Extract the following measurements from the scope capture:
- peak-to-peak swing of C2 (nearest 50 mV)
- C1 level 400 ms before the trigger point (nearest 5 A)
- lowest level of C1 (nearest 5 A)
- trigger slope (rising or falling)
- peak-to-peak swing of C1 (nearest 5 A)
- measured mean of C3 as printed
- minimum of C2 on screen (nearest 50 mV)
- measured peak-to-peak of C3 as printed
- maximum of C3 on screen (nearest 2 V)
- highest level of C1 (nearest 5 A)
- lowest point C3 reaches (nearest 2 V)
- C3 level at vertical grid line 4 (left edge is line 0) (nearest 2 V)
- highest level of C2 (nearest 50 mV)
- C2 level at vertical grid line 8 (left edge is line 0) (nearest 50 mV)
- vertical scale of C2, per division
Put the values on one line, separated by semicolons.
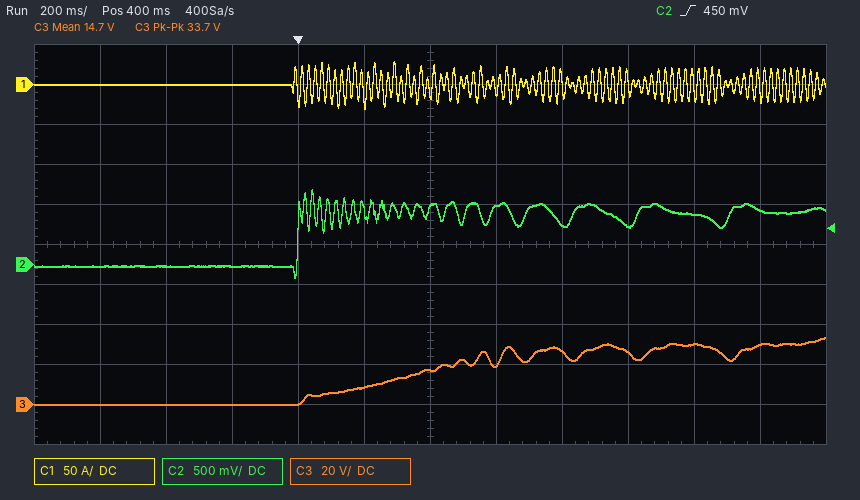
1.10 V; 0 A; -30 A; rising; 60 A; 14.7 V; -150 mV; 33.7 V; 34 V; 30 A; 0 V; 0 V; 950 mV; 500 mV; 500 mV
